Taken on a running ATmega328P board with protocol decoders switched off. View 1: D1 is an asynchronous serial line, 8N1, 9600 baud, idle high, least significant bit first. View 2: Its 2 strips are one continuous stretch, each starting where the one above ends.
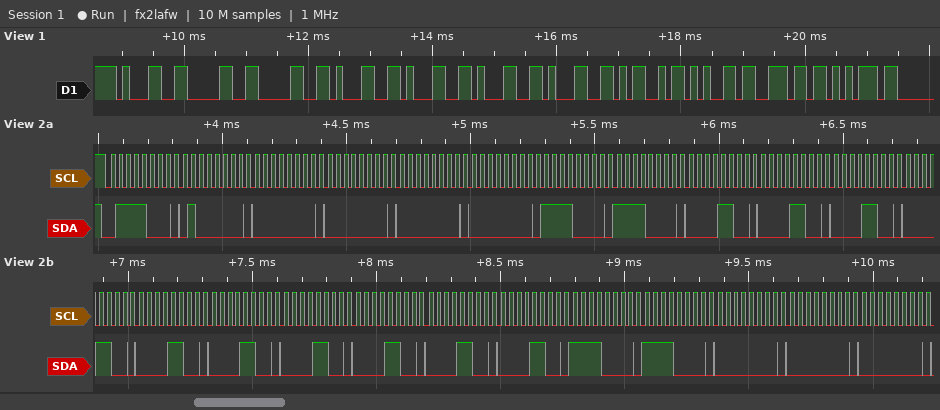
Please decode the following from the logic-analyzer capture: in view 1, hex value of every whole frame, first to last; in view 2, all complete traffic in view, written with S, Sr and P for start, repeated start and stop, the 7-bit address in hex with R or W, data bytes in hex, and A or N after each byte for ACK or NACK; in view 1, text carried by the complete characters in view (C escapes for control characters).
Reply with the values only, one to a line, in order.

0x31 0x30 0x30 0x31 0x31 0x31 0x31 0x4D 0x65 0x6E 0x75
S 3CW A 40 A 00 A 00 A 00 A 00 A F0 A F0 A 0C A 0C A 0C A 0C A 0C A 0C A 0C A 0C A 0C A 0C A F0 A F0 A 00 A 00 A 00 A
"1001111Menu"
